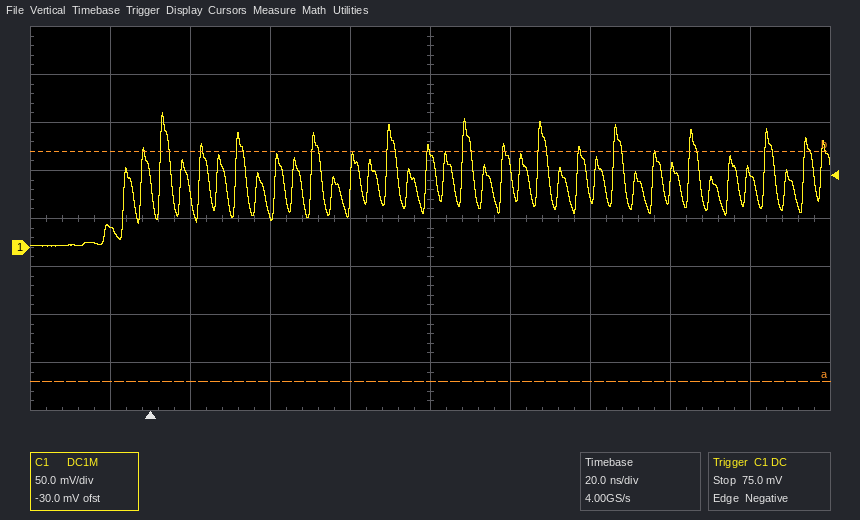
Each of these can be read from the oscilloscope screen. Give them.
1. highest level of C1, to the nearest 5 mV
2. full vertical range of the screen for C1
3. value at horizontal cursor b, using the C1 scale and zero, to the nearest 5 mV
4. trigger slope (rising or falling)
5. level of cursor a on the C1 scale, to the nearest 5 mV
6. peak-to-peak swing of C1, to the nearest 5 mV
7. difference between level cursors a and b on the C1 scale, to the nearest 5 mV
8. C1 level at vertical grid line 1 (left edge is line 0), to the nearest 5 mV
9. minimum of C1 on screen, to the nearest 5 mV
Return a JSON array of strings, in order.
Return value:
["140 mV", "400 mV", "100 mV", "falling", "-140 mV", "140 mV", "240 mV", "20 mV", "0 mV"]
